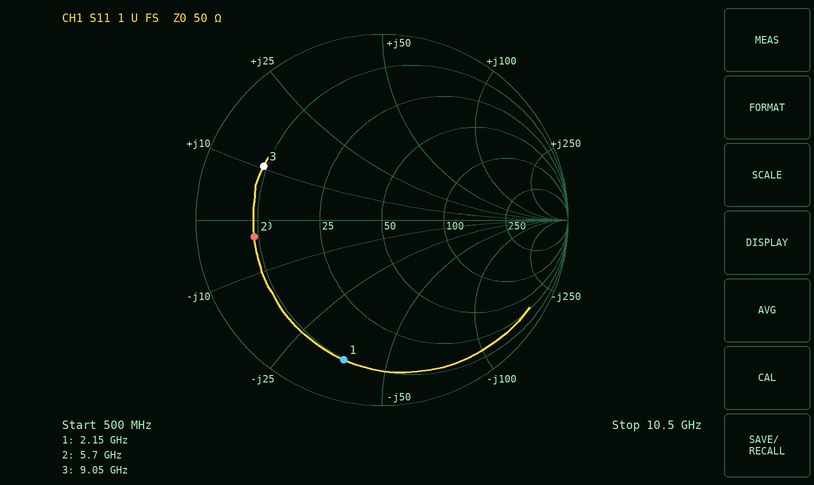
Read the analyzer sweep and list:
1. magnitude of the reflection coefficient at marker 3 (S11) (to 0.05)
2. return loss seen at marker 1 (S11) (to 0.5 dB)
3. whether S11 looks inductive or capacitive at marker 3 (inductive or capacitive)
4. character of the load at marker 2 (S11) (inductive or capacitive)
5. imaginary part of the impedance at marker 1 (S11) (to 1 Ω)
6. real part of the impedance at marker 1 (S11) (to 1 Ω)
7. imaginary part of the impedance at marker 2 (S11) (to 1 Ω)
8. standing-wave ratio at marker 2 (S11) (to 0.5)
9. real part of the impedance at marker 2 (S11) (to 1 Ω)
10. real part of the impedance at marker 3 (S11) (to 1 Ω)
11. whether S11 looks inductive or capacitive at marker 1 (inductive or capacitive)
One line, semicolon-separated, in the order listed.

0.70; 2.0 dB; inductive; capacitive; -37 Ω; 10 Ω; -3 Ω; 5.5; 9 Ω; 9 Ω; capacitive
